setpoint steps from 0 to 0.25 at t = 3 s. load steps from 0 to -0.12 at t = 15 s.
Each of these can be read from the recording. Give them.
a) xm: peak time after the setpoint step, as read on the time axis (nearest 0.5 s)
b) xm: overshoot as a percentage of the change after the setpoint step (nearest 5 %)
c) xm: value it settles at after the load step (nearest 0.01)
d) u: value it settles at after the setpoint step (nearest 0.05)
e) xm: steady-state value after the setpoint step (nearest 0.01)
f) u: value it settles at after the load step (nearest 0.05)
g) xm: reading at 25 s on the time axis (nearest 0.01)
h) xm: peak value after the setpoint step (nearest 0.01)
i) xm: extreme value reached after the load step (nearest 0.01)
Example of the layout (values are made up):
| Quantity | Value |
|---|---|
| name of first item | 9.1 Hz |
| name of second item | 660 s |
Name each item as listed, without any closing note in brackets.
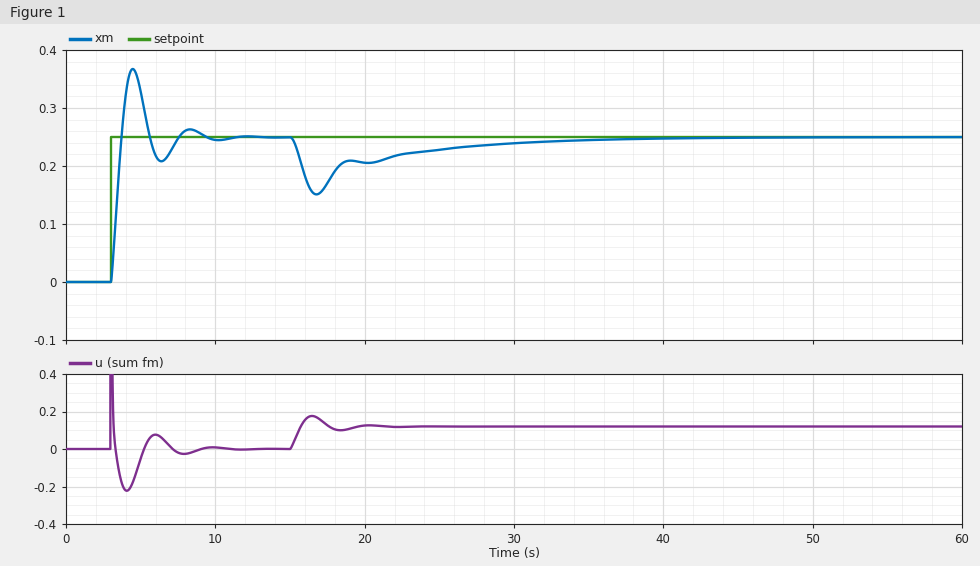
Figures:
| Quantity | Value |
|---|---|
| xm: peak time after the setpoint step, as read on the time axis | 4.5 s |
| xm: overshoot as a percentage of the change after the setpoint step | 45 % |
| xm: value it settles at after the load step | 0.25 |
| u: value it settles at after the setpoint step | 0.00 |
| xm: steady-state value after the setpoint step | 0.25 |
| u: value it settles at after the load step | 0.10 |
| xm: reading at 25 s on the time axis | 0.23 |
| xm: peak value after the setpoint step | 0.37 |
| xm: extreme value reached after the load step | 0.15 |
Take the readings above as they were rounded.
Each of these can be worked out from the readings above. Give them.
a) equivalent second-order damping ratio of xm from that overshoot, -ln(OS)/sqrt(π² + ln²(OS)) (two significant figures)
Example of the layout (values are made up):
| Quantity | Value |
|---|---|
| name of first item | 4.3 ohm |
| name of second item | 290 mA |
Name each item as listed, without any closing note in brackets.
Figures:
| Quantity | Value |
|---|---|
| equivalent second-order damping ratio of xm from that overshoot, -ln(OS)/sqrt(π² + ln²(OS)) | 0.25 |
